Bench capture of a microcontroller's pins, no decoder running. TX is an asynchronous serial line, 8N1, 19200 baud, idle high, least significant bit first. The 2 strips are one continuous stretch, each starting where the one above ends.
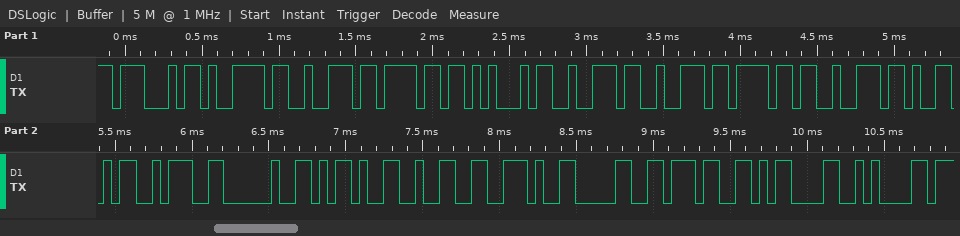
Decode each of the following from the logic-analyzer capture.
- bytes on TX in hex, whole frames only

47 79 72 6F 45 72 72 6F 72 59 3A 20 2D 32 2E 30 37 0D 0A
